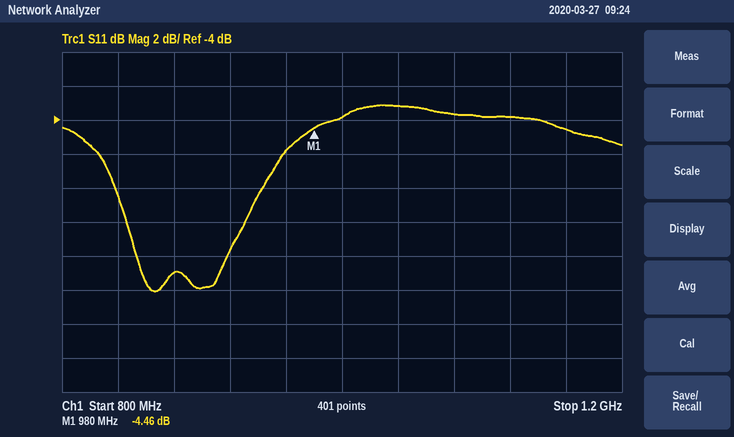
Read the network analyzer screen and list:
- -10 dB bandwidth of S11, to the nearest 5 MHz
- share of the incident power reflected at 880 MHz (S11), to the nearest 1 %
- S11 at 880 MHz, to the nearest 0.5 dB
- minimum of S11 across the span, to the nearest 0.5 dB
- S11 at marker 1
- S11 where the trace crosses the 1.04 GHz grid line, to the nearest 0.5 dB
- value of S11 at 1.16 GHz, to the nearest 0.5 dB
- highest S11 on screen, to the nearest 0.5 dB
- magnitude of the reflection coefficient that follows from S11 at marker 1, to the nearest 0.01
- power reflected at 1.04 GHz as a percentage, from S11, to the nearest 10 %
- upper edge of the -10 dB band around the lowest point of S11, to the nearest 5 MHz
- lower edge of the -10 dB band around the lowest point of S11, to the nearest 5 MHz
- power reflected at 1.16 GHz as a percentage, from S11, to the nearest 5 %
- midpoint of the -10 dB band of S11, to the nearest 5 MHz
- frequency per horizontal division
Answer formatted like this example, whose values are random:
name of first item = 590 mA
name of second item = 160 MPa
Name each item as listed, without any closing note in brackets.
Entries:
-10 dB bandwidth of S11, to the nearest 5 MHz = 85 MHz
share of the incident power reflected at 880 MHz (S11), to the nearest 1 % = 5 %
S11 at 880 MHz, to the nearest 0.5 dB = -13.0 dB
minimum of S11 across the span, to the nearest 0.5 dB = -14.0 dB
S11 at marker 1 = -4.46 dB
S11 where the trace crosses the 1.04 GHz grid line, to the nearest 0.5 dB = -3.0 dB
value of S11 at 1.16 GHz, to the nearest 0.5 dB = -4.5 dB
highest S11 on screen, to the nearest 0.5 dB = -3.0 dB
magnitude of the reflection coefficient that follows from S11 at marker 1, to the nearest 0.01 = 0.60
power reflected at 1.04 GHz as a percentage, from S11, to the nearest 10 % = 50 %
upper edge of the -10 dB band around the lowest point of S11, to the nearest 5 MHz = 930 MHz
lower edge of the -10 dB band around the lowest point of S11, to the nearest 5 MHz = 845 MHz
power reflected at 1.16 GHz as a percentage, from S11, to the nearest 5 % = 35 %
midpoint of the -10 dB band of S11, to the nearest 5 MHz = 890 MHz
frequency per horizontal division = 40 MHz
